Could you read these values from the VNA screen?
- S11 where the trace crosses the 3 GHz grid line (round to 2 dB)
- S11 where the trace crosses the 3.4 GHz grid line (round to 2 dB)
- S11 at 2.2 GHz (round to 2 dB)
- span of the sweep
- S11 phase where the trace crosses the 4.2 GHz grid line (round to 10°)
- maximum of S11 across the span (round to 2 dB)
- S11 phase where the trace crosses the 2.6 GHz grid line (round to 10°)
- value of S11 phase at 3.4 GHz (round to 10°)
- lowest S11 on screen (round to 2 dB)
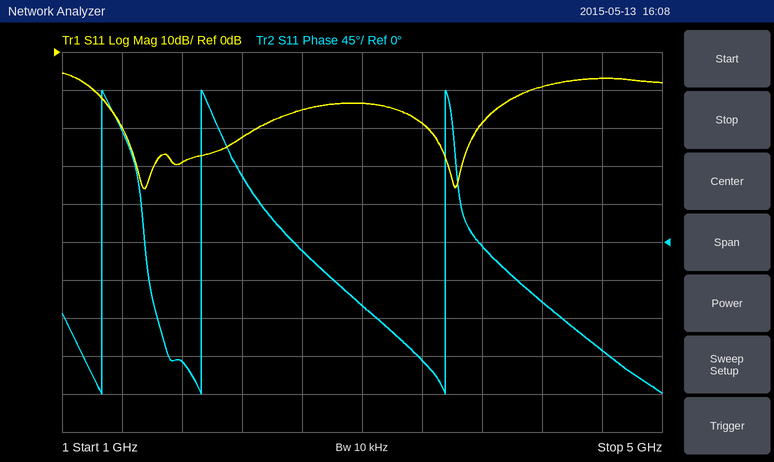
-14 dB
-18 dB
-22 dB
4 GHz
-70°
-6 dB
-10°
-140°
-36 dB
